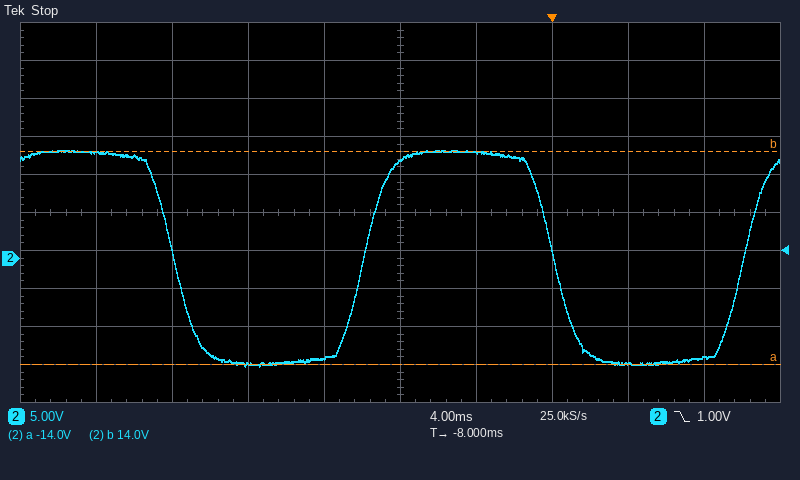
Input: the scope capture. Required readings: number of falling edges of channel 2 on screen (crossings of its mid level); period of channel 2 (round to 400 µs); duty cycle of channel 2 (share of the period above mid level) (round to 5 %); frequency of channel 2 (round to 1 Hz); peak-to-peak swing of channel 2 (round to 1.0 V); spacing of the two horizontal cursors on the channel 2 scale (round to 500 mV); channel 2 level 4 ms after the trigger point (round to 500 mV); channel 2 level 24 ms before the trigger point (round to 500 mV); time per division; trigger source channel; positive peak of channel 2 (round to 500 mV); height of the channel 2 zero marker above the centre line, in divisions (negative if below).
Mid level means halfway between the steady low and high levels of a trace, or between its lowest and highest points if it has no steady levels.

2
20.0 ms
50 %
50 Hz
28.0 V
28.0 V
-14.0 V
14.0 V
4 ms
channel 2
14.0 V
-1.2 div
